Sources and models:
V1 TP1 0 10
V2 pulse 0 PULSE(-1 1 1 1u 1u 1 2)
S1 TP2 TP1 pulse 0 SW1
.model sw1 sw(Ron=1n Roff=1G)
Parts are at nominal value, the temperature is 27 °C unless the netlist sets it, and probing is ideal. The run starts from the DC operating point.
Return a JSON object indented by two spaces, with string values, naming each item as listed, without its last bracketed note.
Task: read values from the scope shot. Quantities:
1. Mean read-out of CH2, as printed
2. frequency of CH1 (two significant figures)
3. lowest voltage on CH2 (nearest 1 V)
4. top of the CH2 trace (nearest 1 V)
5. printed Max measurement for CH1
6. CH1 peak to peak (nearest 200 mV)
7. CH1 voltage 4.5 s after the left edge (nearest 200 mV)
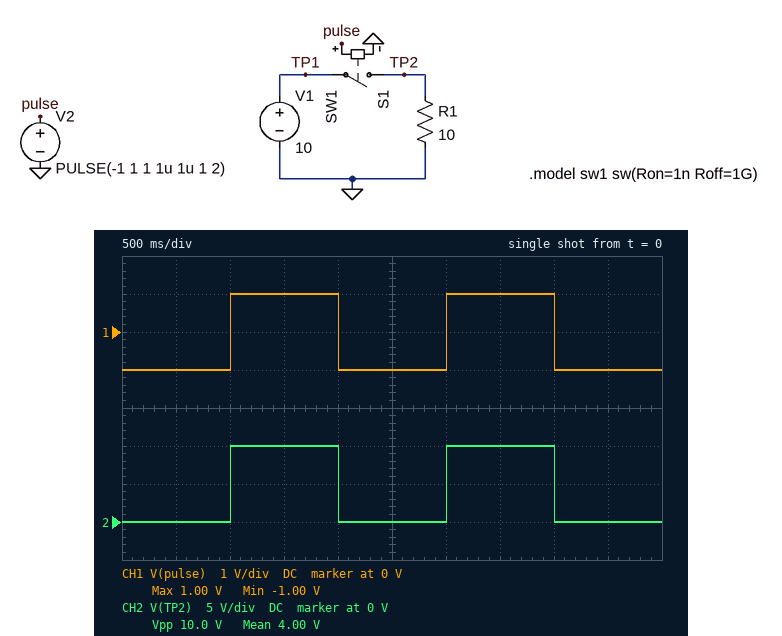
{
  "Mean read-out of CH2, as printed": "4.00 V",
  "frequency of CH1": "500 mHz",
  "lowest voltage on CH2": "0 V",
  "top of the CH2 trace": "10 V",
  "printed Max measurement for CH1": "1.00 V",
  "CH1 peak to peak": "2.0 V",
  "CH1 voltage 4.5 s after the left edge": "-1.0 V"
}
